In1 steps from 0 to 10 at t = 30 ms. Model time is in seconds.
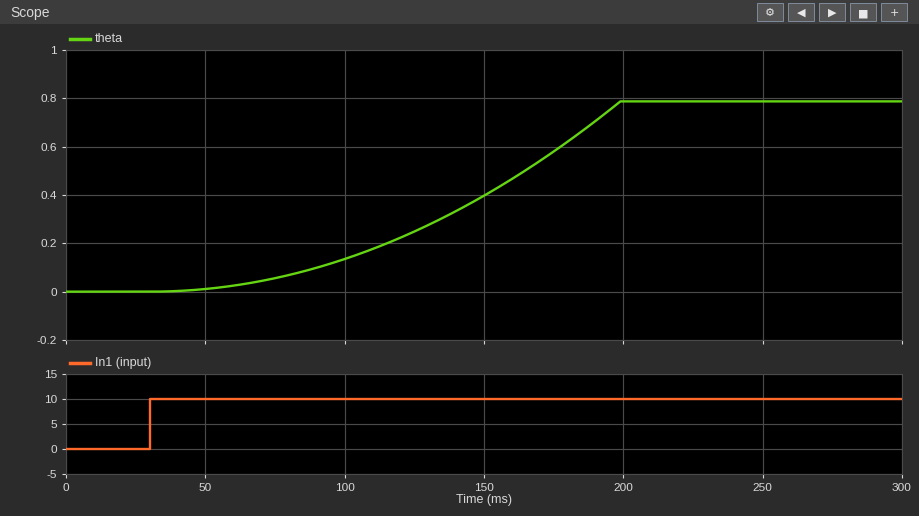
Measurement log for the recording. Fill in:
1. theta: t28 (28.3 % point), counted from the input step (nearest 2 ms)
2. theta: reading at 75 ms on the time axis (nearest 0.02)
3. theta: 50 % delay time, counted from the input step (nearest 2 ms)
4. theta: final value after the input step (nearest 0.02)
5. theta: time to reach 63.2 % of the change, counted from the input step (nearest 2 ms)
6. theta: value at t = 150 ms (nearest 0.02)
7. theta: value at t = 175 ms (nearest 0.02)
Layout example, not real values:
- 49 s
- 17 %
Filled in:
- 90 ms
- 0.06
- 120 ms
- 0.78
- 134 ms
- 0.40
- 0.58
